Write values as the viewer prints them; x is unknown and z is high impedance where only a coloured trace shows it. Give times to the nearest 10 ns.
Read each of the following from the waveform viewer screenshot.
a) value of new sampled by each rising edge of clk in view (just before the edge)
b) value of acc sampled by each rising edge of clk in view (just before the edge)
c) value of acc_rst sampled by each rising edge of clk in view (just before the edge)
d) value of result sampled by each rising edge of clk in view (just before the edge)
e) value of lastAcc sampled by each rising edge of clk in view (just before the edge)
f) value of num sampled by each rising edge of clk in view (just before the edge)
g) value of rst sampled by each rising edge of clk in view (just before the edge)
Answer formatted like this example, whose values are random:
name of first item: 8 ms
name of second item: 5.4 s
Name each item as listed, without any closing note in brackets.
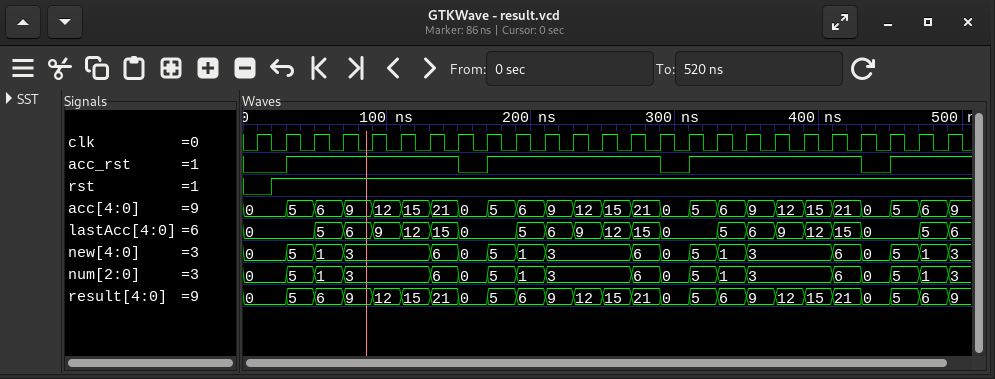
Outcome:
value of new sampled by each rising edge of clk in view: 0, 0, 5, 1, 3, 3, 3, 6, 0, 5, 1, 3, 3, 3, 6, 0, 5, 1, 3, 3, 3, 6, 0, 5, 1
value of acc sampled by each rising edge of clk in view: 0, 0, 5, 6, 9, 12, 15, 21, 0, 5, 6, 9, 12, 15, 21, 0, 5, 6, 9, 12, 15, 21, 0, 5, 6
value of acc_rst sampled by each rising edge of clk in view: 0 0 1 1 1 1 1 1 0 1 1 1 1 1 1 0 1 1 1 1 1 1 0 1 1
value of result sampled by each rising edge of clk in view: 0, 0, 5, 6, 9, 12, 15, 21, 0, 5, 6, 9, 12, 15, 21, 0, 5, 6, 9, 12, 15, 21, 0, 5, 6
value of lastAcc sampled by each rising edge of clk in view: 0, 0, 0, 5, 6, 9, 12, 15, 0, 0, 5, 6, 9, 12, 15, 0, 0, 5, 6, 9, 12, 15, 0, 0, 5
value of num sampled by each rising edge of clk in view: 0, 0, 5, 1, 3, 3, 3, 6, 0, 5, 1, 3, 3, 3, 6, 0, 5, 1, 3, 3, 3, 6, 0, 5, 1
value of rst sampled by each rising edge of clk in view: 0 1 1 1 1 1 1 1 1 1 1 1 1 1 1 1 1 1 1 1 1 1 1 1 1
